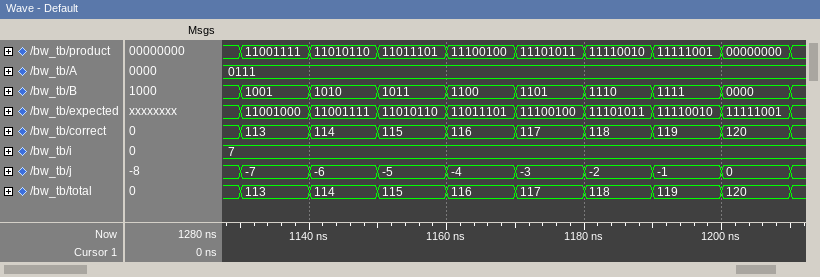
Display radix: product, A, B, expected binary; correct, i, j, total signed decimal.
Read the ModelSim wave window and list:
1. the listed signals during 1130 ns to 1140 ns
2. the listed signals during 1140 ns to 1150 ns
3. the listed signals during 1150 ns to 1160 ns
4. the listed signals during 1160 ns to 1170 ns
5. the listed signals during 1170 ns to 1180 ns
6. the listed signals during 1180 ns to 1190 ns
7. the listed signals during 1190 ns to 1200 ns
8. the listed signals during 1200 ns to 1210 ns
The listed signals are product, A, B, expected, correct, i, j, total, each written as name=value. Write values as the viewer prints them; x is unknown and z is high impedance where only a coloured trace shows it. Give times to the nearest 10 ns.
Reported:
product=11001111, A=0111, B=1001, expected=11001000, correct=113, i=7, j=-7, total=113
product=11010110, A=0111, B=1010, expected=11001111, correct=114, i=7, j=-6, total=114
product=11011101, A=0111, B=1011, expected=11010110, correct=115, i=7, j=-5, total=115
product=11100100, A=0111, B=1100, expected=11011101, correct=116, i=7, j=-4, total=116
product=11101011, A=0111, B=1101, expected=11100100, correct=117, i=7, j=-3, total=117
product=11110010, A=0111, B=1110, expected=11101011, correct=118, i=7, j=-2, total=118
product=11111001, A=0111, B=1111, expected=11110010, correct=119, i=7, j=-1, total=119
product=00000000, A=0111, B=0000, expected=11111001, correct=120, i=7, j=0, total=120
